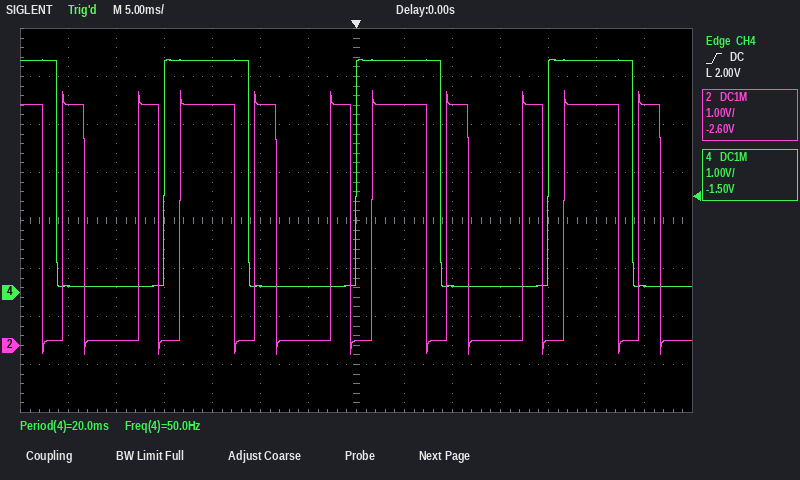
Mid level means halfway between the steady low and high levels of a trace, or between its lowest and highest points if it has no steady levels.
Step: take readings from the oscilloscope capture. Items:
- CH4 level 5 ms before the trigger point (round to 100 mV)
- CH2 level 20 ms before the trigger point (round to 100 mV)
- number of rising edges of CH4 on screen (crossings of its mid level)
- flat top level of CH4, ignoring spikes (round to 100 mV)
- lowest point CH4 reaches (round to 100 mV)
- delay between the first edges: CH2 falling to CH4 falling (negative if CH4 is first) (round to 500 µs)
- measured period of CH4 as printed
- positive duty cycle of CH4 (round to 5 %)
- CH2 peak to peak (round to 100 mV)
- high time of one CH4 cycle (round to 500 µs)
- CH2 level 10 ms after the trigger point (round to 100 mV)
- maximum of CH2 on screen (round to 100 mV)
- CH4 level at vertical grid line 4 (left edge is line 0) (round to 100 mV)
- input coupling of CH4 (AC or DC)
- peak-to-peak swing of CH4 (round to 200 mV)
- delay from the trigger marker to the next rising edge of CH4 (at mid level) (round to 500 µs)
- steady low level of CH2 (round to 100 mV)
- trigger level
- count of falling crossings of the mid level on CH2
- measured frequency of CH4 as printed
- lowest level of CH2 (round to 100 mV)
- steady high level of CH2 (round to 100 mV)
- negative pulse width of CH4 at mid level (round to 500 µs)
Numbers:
100 mV
100 mV
3
4.8 V
100 mV
+1.5 ms
20.0 ms
45 %
5.5 V
9.0 ms
5.0 V
5.3 V
4.8 V
DC
4.8 V
20.0 ms
100 mV
2.00 V
11
50.0 Hz
-200 mV
5.0 V
11.0 ms
